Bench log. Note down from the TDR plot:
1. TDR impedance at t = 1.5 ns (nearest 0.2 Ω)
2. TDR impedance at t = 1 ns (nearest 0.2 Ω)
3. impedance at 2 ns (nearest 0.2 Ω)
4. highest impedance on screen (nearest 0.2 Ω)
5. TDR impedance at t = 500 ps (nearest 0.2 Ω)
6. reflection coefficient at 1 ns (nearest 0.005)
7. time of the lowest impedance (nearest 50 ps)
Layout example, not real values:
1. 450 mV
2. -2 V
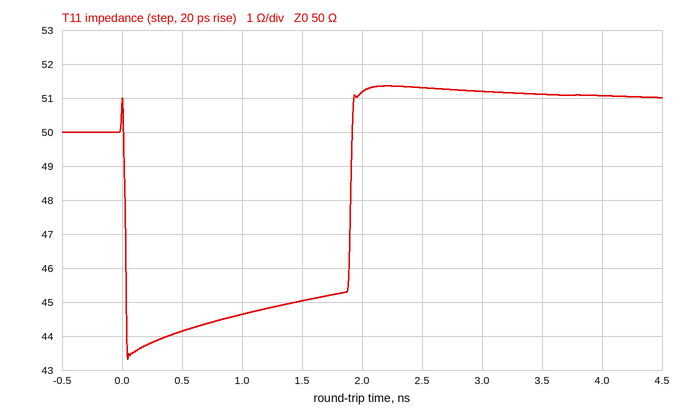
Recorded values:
1. 45.0 Ω
2. 44.6 Ω
3. 51.2 Ω
4. 51.4 Ω
5. 44.2 Ω
6. -0.055
7. 50 ps
